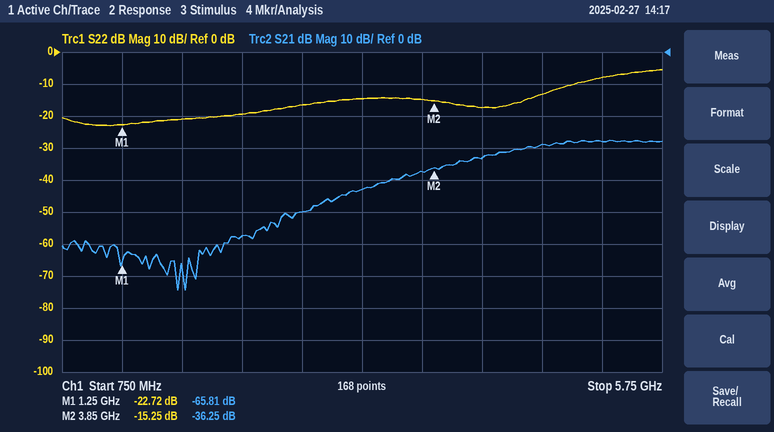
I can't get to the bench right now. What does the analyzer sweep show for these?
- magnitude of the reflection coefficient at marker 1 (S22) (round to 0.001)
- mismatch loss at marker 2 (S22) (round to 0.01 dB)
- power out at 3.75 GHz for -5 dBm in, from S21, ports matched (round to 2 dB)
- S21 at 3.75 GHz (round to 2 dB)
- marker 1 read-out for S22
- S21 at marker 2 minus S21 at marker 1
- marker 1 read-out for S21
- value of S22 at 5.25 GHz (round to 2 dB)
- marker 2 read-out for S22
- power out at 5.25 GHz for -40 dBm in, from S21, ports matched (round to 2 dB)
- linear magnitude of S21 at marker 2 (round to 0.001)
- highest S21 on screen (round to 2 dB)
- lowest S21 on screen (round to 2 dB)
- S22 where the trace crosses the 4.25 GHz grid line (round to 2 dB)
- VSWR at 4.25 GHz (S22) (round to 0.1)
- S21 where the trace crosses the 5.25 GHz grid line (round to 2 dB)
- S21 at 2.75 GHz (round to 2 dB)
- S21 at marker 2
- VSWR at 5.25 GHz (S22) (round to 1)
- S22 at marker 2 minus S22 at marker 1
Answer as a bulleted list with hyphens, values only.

- 0.073
- 0.13 dB
- -42 dBm
- -38 dB
- -22.72 dB
- 29.56 dB
- -65.81 dB
- -8 dB
- -15.25 dB
- -68 dBm
- 0.015
- -28 dB
- -74 dB
- -18 dB
- 1.3
- -28 dB
- -50 dB
- -36.25 dB
- 2
- 7.47 dB
